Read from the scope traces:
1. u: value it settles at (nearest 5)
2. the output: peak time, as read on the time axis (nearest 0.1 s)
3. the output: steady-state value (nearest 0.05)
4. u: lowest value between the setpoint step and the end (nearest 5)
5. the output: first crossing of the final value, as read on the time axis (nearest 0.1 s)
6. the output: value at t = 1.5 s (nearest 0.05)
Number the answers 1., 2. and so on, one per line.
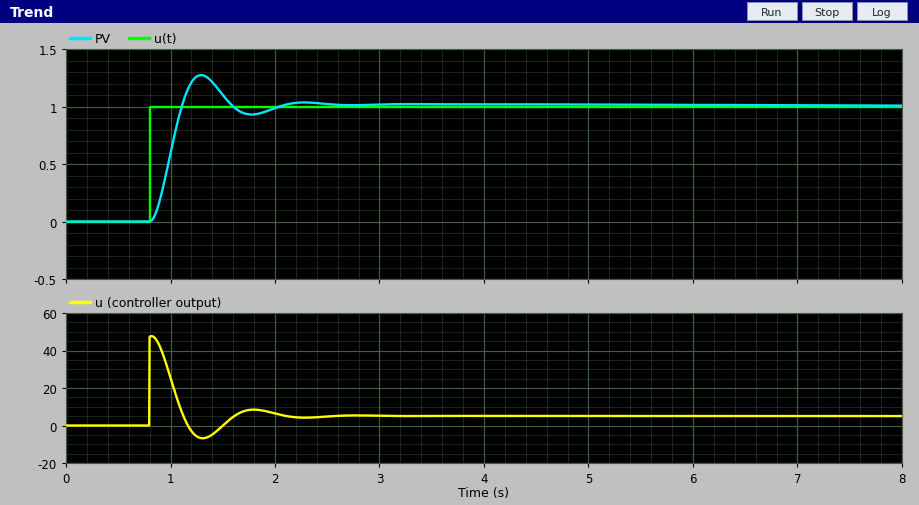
1. 5
2. 1.3 s
3. 1.00
4. -5
5. 1.1 s
6. 1.10
